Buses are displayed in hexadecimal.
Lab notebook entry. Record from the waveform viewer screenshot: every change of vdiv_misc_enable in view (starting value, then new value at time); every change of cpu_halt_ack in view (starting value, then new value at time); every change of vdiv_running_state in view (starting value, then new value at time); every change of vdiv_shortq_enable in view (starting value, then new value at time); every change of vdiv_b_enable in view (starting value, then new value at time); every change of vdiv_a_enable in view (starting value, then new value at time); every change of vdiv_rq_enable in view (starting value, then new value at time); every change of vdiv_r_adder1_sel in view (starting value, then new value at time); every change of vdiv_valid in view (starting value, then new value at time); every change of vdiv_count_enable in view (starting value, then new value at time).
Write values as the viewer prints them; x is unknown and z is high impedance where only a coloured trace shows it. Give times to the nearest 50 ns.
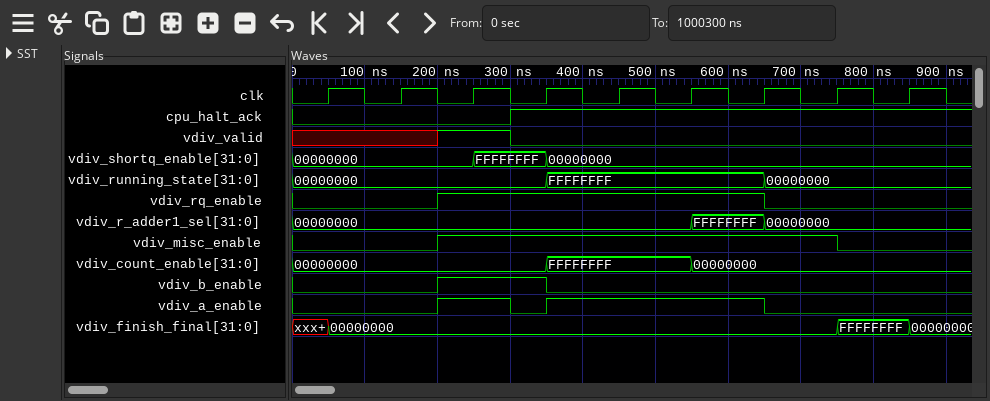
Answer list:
0, 1 at 200 ns, 0 at 750 ns
0, 1 at 300 ns
00000000, FFFFFFFF at 350 ns, 00000000 at 650 ns
00000000, FFFFFFFF at 250 ns, 00000000 at 350 ns
0, 1 at 200 ns, 0 at 350 ns
0, 1 at 200 ns, 0 at 300 ns, 1 at 350 ns, 0 at 650 ns
0, 1 at 200 ns, 0 at 650 ns
00000000, FFFFFFFF at 550 ns, 00000000 at 650 ns
x, 1 at 200 ns, 0 at 300 ns
00000000, FFFFFFFF at 350 ns, 00000000 at 550 ns
